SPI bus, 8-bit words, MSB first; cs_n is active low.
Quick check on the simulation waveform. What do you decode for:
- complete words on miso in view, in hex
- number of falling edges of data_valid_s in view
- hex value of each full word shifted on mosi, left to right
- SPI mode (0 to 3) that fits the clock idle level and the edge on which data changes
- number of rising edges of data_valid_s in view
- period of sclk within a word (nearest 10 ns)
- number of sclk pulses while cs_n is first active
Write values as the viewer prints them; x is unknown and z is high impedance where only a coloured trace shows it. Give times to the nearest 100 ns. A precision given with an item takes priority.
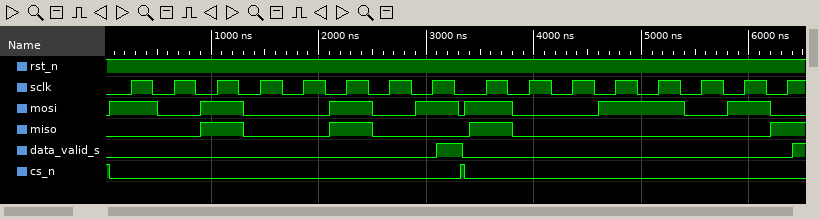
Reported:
24, 81
1
A5, 9A
0
2
400 ns
8
